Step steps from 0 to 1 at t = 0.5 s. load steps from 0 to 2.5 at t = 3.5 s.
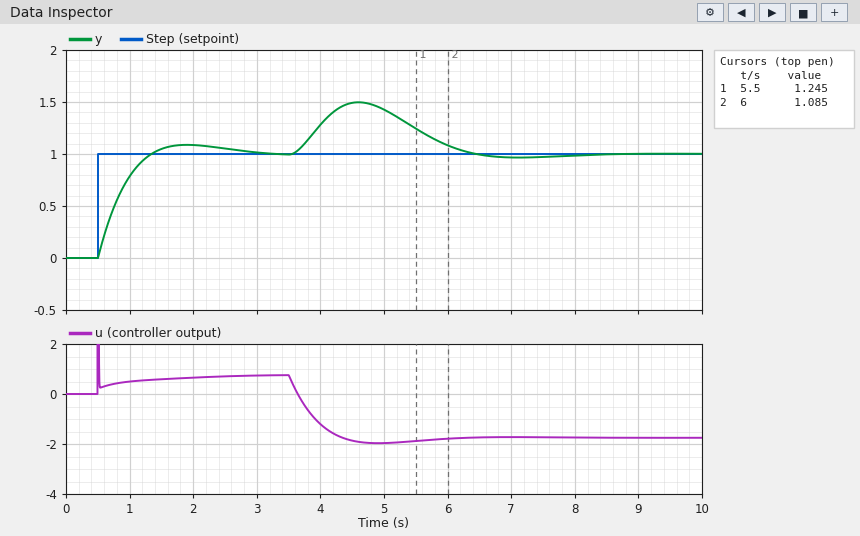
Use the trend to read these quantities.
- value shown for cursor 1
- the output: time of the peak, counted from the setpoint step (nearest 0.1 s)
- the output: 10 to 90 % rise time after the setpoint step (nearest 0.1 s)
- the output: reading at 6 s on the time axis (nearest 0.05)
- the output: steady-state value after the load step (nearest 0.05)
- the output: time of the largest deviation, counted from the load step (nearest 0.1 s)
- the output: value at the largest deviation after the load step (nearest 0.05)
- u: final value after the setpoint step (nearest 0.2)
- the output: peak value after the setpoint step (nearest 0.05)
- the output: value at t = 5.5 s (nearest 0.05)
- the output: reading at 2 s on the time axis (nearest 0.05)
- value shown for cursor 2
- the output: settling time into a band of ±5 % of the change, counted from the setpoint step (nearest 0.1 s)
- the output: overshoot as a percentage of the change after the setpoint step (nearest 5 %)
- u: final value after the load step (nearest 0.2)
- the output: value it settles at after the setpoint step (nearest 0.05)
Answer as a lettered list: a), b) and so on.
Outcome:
a) 1.245
b) 1.4 s
c) 0.6 s
d) 1.10
e) 1.00
f) 1.1 s
g) 1.50
h) 0.8
i) 1.10
j) 1.25
k) 1.10
l) 1.085
m) 2.0 s
n) 10 %
o) -1.8
p) 1.00
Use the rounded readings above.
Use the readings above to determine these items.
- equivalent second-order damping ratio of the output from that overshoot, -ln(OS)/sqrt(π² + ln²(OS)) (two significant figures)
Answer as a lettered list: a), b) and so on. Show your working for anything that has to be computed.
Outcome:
a) ln(0.1) = -2.303; 2.303 / sqrt(9.870 + 5.302) = 0.59
